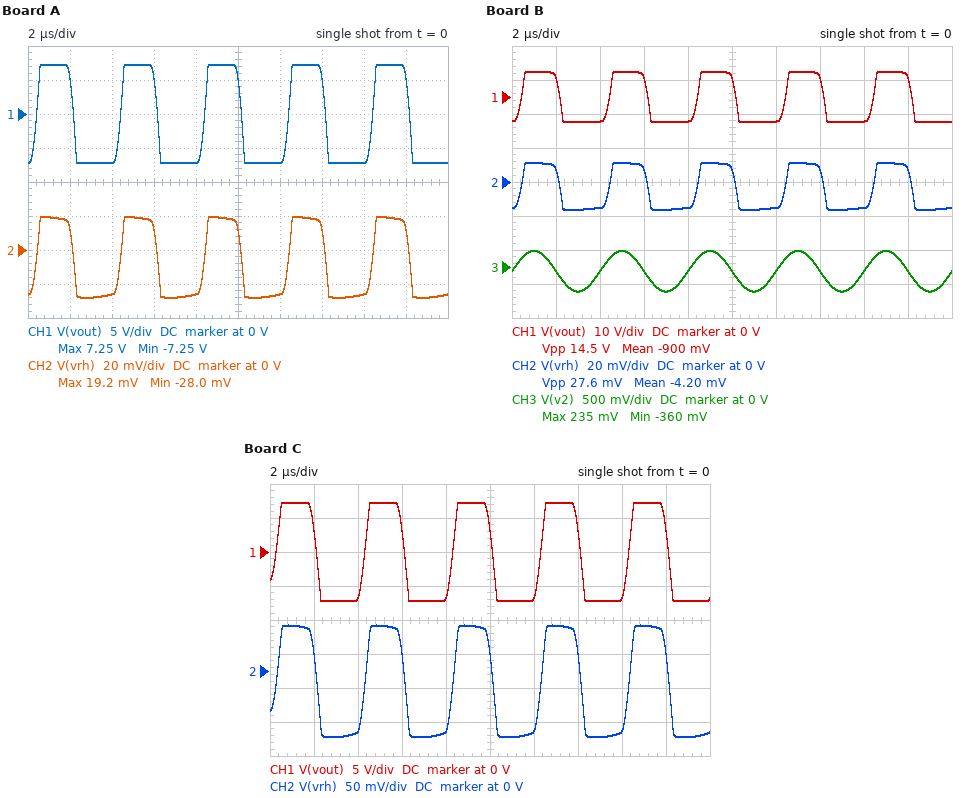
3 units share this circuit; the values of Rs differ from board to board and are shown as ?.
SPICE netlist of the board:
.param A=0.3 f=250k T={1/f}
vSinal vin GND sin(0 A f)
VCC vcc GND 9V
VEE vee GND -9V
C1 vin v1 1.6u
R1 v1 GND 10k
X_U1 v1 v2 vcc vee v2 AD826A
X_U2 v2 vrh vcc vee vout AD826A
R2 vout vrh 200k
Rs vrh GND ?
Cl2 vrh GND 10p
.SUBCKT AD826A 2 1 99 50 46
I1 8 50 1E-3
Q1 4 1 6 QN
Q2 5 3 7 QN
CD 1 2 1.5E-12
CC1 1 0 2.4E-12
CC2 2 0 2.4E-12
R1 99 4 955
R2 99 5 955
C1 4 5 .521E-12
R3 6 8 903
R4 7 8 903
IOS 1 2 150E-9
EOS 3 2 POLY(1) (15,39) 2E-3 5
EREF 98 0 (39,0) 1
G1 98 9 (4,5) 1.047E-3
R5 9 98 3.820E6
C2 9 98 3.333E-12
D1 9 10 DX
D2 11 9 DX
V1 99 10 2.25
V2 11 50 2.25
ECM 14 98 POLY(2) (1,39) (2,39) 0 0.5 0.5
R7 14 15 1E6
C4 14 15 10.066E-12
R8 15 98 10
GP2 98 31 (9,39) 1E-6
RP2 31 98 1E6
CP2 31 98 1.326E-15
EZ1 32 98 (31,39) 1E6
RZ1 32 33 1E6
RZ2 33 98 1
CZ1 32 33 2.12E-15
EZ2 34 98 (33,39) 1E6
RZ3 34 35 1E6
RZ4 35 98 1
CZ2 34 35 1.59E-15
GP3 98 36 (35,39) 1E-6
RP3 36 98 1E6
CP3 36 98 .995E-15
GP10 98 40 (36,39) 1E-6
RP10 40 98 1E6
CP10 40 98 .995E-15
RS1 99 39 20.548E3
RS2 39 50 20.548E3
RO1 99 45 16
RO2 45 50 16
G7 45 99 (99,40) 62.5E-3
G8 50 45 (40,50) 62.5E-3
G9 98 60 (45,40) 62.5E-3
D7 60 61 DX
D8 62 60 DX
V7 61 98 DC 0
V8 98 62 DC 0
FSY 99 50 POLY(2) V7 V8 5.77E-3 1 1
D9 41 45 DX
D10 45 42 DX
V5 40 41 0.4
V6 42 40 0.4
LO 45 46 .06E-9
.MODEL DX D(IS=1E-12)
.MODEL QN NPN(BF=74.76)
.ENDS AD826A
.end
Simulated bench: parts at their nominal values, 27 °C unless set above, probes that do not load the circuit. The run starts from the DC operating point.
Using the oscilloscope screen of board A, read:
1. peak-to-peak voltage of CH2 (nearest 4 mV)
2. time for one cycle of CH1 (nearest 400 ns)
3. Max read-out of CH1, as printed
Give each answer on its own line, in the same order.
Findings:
48 mV
4.0 µs
7.25 V
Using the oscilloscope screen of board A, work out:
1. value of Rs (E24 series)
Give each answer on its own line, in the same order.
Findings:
620 Ω
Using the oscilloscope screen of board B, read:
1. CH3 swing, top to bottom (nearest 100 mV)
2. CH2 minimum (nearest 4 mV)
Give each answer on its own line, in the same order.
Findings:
600 mV
-16 mV
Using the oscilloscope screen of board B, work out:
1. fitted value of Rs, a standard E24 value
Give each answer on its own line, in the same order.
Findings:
360 Ω
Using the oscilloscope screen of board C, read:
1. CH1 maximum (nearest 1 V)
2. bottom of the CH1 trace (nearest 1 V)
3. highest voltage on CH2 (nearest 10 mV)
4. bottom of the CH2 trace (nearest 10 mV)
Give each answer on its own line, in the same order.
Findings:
7 V
-7 V
70 mV
-100 mV
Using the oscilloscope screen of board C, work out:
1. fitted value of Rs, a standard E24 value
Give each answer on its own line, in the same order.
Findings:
2.2 kΩ
